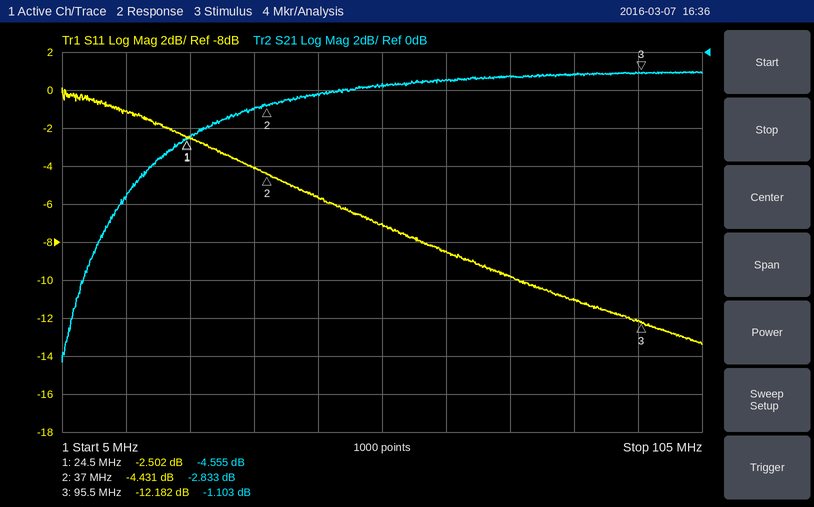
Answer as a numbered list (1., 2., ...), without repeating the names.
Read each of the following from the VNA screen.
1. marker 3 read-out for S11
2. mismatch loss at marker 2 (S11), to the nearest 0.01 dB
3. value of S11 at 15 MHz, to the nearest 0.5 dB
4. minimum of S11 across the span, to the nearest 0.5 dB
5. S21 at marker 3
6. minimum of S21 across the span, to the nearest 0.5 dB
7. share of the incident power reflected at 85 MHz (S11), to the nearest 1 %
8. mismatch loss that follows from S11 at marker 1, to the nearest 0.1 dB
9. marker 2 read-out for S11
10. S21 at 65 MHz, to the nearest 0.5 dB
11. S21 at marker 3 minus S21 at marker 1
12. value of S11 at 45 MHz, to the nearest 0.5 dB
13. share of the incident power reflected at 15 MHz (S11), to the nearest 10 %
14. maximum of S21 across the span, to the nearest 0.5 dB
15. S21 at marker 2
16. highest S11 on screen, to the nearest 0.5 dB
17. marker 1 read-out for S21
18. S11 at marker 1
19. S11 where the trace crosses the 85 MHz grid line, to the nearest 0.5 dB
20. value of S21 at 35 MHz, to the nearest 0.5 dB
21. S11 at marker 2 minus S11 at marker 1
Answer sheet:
1. -12.182 dB
2. 1.94 dB
3. -1.0 dB
4. -13.5 dB
5. -1.103 dB
6. -16.5 dB
7. 8 %
8. 3.6 dB
9. -4.431 dB
10. -1.5 dB
11. 3.452 dB
12. -5.5 dB
13. 80 %
14. -1.0 dB
15. -2.833 dB
16. 0.0 dB
17. -4.555 dB
18. -2.502 dB
19. -11.0 dB
20. -3.0 dB
21. -1.929 dB
